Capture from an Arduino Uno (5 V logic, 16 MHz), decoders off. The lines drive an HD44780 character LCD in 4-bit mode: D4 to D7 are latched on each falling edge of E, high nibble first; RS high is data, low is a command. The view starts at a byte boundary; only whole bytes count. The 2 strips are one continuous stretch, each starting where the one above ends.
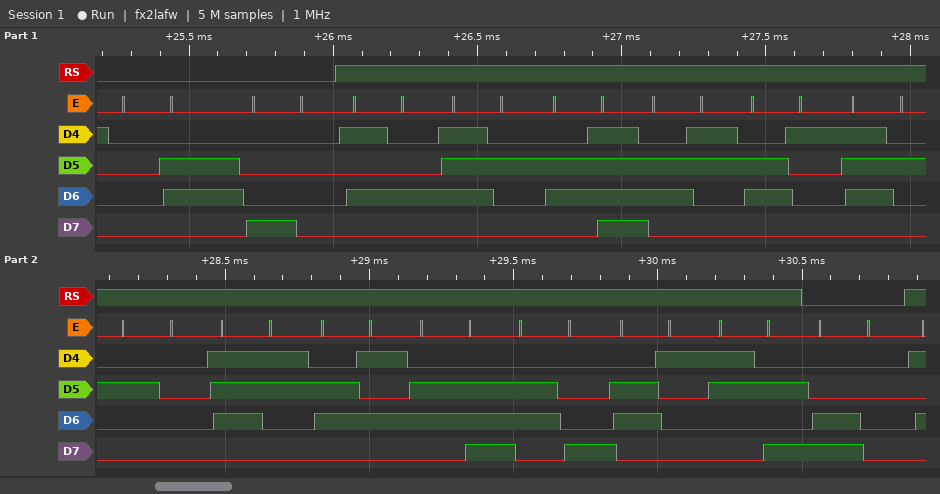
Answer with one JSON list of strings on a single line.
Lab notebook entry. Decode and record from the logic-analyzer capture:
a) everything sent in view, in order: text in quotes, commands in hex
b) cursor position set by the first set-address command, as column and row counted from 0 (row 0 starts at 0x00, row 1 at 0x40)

["0x06 0x80 \"Trocar senha:\" 0xC0", "column 0, row 0"]
